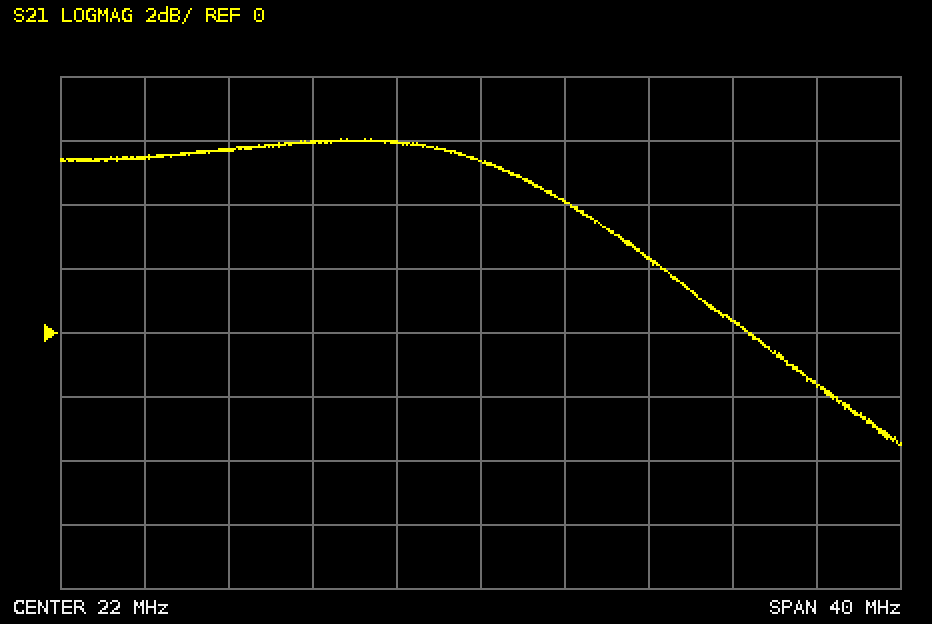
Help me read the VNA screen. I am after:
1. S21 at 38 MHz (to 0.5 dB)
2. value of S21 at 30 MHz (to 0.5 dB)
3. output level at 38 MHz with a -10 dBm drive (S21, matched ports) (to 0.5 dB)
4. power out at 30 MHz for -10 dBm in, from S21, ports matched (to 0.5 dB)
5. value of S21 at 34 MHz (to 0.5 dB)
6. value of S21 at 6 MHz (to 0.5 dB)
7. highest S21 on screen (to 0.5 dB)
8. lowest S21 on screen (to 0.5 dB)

-1.5 dB
2.5 dB
-11.5 dBm
-7.5 dBm
0.5 dB
5.5 dB
6.0 dB
-3.5 dB
